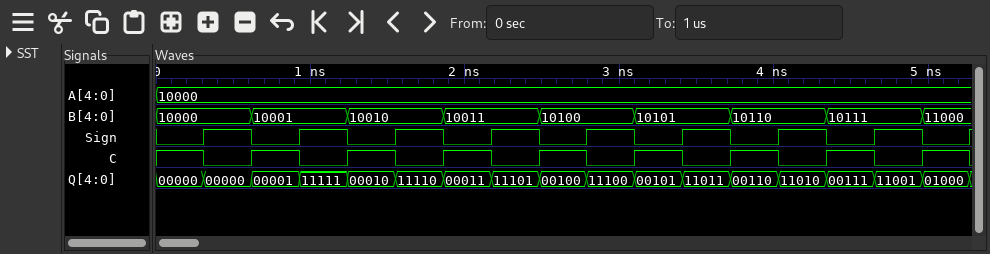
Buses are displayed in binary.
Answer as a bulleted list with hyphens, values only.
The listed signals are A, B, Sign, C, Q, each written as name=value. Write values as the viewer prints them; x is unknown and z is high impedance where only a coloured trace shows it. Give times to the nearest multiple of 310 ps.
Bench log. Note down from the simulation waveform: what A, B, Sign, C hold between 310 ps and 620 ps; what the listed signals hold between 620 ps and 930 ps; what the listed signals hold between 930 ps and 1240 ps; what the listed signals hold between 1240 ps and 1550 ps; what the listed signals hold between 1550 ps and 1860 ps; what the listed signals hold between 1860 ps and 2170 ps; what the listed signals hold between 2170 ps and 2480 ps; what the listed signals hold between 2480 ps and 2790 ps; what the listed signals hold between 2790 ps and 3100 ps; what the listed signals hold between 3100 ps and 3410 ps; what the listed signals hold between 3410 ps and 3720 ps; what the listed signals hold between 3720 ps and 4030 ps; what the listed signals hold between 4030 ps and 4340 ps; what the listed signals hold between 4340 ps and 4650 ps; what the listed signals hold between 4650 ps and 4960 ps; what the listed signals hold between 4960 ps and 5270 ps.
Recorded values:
- A=10000, B=10000, Sign=1, C=0
- A=10000, B=10001, Sign=0, C=1, Q=00001
- A=10000, B=10001, Sign=1, C=0, Q=11111
- A=10000, B=10010, Sign=0, C=1, Q=00010
- A=10000, B=10010, Sign=1, C=0, Q=11110
- A=10000, B=10011, Sign=0, C=1, Q=00011
- A=10000, B=10011, Sign=1, C=0, Q=11101
- A=10000, B=10100, Sign=0, C=1, Q=00100
- A=10000, B=10100, Sign=1, C=0, Q=11100
- A=10000, B=10101, Sign=0, C=1, Q=00101
- A=10000, B=10101, Sign=1, C=0, Q=11011
- A=10000, B=10110, Sign=0, C=1, Q=00110
- A=10000, B=10110, Sign=1, C=0, Q=11010
- A=10000, B=10111, Sign=0, C=1, Q=00111
- A=10000, B=10111, Sign=1, C=0, Q=11001
- A=10000, B=11000, Sign=0, C=1, Q=01000
